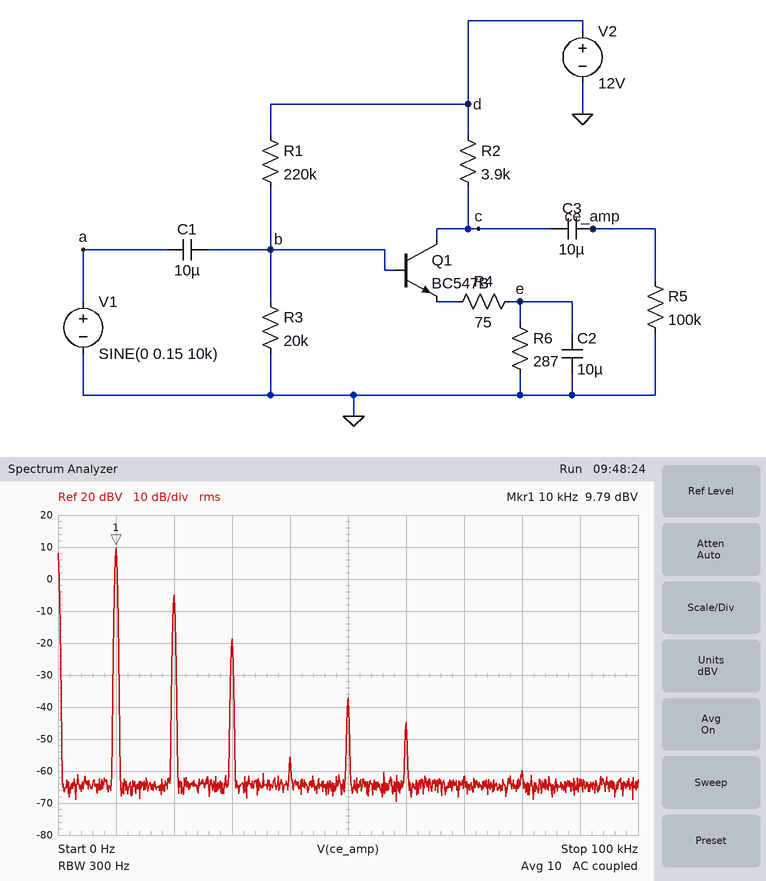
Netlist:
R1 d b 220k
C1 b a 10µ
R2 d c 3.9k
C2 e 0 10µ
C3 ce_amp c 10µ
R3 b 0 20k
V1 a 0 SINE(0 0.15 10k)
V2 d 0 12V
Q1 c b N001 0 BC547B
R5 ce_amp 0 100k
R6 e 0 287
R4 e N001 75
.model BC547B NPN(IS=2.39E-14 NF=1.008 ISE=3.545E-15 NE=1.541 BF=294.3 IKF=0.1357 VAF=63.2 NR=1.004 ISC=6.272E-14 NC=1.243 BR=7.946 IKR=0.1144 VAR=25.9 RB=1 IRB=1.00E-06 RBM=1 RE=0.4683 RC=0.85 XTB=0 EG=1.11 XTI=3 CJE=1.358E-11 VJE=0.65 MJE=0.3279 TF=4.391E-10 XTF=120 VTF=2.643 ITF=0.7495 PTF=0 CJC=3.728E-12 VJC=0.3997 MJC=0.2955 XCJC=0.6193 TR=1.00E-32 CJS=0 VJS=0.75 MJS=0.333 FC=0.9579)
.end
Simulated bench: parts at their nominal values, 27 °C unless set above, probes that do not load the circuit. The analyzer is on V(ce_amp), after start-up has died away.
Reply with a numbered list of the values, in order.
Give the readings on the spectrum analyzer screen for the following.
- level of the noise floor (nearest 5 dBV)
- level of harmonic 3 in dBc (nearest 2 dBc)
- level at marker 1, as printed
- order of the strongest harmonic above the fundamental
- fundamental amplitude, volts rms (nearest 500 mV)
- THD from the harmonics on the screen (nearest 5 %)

1. -65 dBV
2. -28 dBc
3. 9.79 dBV
4. 2
5. 3.0 V
6. 20 %
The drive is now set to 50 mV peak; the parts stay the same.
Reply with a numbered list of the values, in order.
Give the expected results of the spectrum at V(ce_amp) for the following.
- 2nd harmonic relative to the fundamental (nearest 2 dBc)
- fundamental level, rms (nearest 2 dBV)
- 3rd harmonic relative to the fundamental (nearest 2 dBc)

1. -28 dBc
2. 2 dBV
3. -48 dBc
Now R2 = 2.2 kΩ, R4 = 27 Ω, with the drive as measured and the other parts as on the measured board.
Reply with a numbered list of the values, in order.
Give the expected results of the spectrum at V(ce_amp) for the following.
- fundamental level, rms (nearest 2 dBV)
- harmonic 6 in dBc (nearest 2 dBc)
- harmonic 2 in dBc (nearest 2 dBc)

1. 8 dBV
2. -44 dBc
3. -8 dBc
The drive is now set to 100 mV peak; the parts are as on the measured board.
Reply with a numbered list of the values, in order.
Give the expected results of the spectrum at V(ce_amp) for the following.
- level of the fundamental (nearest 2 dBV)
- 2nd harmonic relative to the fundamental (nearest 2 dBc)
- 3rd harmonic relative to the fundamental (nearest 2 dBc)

1. 8 dBV
2. -20 dBc
3. -34 dBc
